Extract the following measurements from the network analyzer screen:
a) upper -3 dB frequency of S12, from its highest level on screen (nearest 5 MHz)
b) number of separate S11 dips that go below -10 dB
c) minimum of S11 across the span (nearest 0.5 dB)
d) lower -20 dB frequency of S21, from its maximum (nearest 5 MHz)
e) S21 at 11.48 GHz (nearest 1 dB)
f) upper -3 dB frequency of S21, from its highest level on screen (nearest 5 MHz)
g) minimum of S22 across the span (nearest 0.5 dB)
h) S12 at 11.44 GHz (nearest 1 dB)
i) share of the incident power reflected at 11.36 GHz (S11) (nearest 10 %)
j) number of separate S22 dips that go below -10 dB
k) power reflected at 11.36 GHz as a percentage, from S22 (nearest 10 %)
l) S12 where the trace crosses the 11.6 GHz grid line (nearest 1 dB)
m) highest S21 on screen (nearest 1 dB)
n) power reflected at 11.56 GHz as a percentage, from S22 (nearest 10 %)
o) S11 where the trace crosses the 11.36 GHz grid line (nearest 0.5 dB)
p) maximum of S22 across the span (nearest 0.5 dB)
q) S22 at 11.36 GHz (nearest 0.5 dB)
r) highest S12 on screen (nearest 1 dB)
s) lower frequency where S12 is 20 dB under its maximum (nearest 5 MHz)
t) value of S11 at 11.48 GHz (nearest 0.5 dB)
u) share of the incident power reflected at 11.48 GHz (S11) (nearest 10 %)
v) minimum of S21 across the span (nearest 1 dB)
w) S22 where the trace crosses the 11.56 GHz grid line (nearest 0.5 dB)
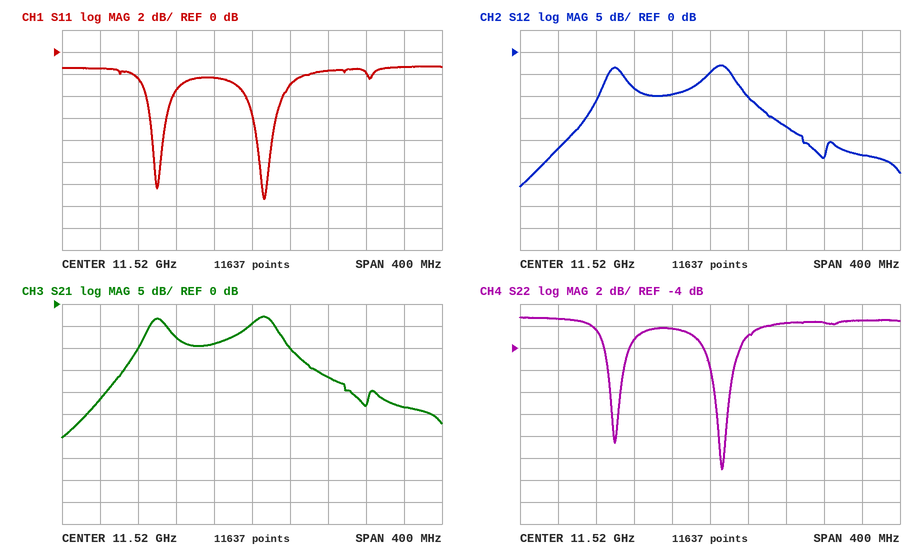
11.545 GHz
2
-13.5 dB
11.355 GHz
-9 dB
11.545 GHz
-15.0 dB
-8 dB
70 %
2
70 %
-17 dB
-3 dB
50 %
-1.5 dB
-1.0 dB
-1.5 dB
-3 dB
11.355 GHz
-2.5 dB
60 %
-30 dB
-3.0 dB
